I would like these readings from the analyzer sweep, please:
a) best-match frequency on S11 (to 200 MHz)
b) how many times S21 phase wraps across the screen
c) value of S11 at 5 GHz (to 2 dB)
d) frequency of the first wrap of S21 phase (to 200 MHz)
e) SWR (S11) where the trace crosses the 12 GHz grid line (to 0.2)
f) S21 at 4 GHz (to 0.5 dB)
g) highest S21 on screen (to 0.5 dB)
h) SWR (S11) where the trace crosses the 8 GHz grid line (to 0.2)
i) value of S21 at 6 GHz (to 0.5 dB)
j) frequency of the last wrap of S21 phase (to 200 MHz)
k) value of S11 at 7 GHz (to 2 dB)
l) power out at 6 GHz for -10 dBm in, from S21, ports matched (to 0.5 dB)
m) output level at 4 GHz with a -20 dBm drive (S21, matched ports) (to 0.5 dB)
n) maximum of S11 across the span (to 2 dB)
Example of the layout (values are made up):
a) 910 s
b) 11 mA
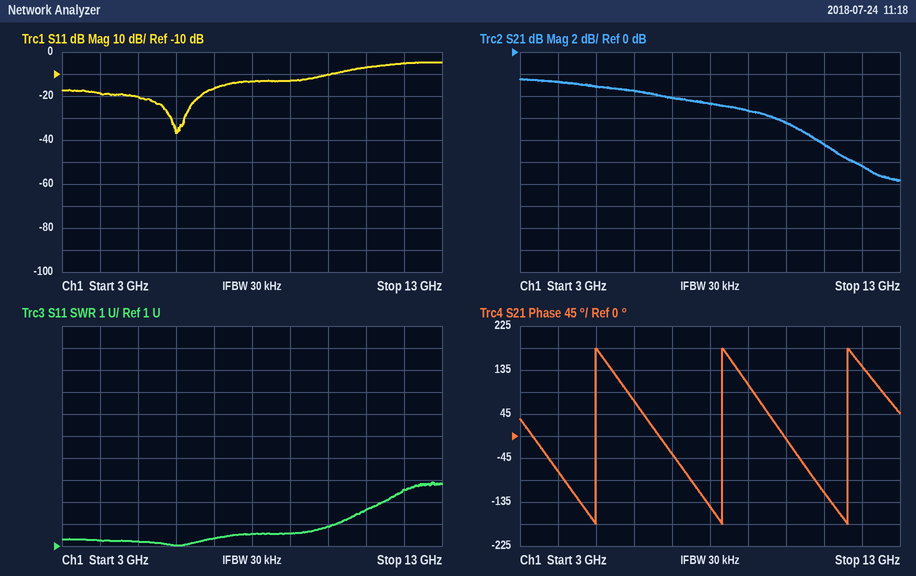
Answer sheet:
a) 6.0 GHz
b) 3
c) -20 dB
d) 5.0 GHz
e) 3.6
f) -2.5 dB
g) -2.5 dB
h) 1.6
i) -3.5 dB
j) 11.6 GHz
k) -16 dB
l) -13.5 dBm
m) -22.5 dBm
n) -4 dB
